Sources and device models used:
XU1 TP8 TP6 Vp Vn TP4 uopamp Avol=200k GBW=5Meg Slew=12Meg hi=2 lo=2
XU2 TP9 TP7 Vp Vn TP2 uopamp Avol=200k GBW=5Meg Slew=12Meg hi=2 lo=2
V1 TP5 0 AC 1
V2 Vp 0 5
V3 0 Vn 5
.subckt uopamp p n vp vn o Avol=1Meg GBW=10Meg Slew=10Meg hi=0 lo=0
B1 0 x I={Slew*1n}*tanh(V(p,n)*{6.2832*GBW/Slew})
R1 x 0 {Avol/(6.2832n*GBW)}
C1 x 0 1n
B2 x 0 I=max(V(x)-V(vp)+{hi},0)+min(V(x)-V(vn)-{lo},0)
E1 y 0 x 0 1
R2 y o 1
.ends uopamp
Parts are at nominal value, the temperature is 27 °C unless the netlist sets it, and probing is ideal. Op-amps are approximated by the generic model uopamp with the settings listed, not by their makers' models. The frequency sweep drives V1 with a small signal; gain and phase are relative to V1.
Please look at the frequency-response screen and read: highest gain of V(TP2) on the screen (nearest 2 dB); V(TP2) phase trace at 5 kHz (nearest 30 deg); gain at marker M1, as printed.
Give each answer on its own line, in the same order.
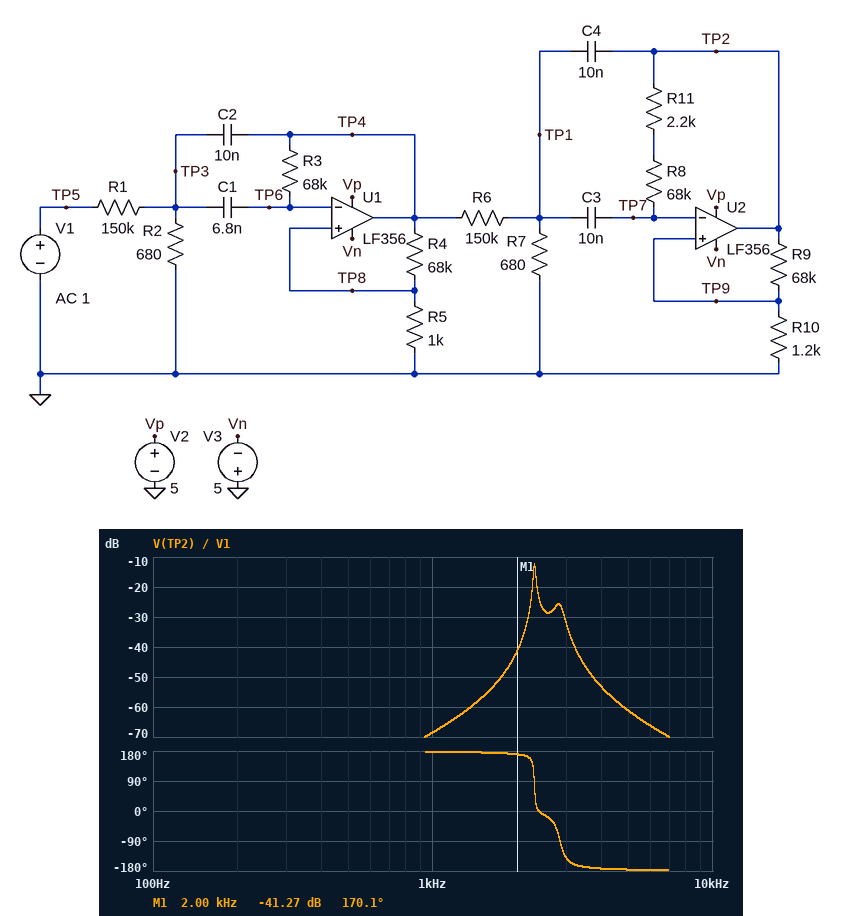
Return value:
-12 dB
-180 deg
-41.27 dB
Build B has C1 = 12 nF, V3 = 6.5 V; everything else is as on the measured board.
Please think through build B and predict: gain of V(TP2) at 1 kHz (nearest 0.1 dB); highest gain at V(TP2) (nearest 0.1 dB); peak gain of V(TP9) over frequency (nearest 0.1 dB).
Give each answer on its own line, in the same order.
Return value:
-62.5 dB
-0.9 dB
-36.1 dB
